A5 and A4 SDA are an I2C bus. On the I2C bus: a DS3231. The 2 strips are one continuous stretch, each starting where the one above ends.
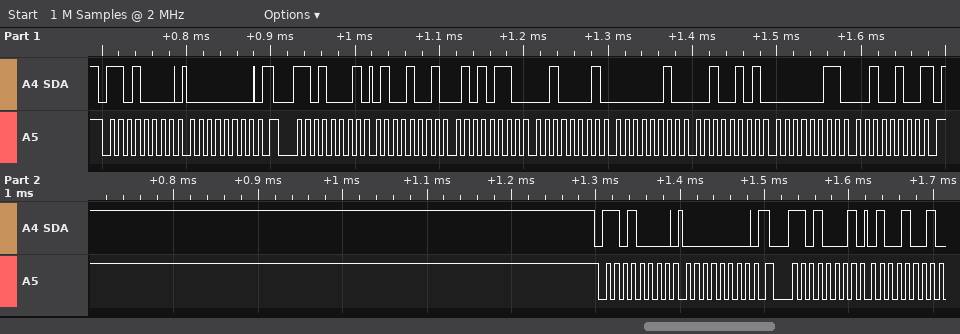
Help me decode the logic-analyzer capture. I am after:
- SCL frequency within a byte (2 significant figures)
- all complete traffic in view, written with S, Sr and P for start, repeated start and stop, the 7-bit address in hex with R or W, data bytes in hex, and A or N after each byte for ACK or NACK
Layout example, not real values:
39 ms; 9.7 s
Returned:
100 kHz; S 68W A 00 A Sr 68R A 49 A 56 A 21 A 02 A 25 A 03 A 24 N P S 68W A 00 A Sr 68R A 49 A
